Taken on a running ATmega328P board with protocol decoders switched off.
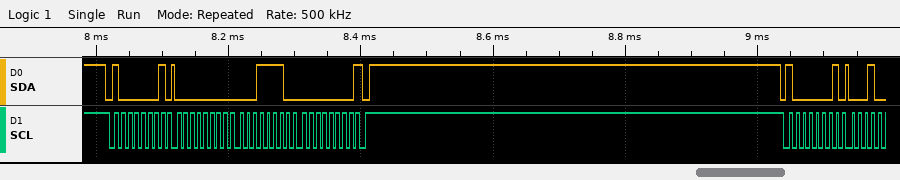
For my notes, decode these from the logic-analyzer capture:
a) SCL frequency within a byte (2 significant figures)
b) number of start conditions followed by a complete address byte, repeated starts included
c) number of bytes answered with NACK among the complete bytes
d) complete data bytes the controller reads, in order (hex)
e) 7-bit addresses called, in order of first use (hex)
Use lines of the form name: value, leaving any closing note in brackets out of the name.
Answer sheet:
SCL frequency within a byte: 100 kHz
number of start conditions followed by a complete address byte, repeated starts included: 2
number of bytes answered with NACK among the complete bytes: 1
complete data bytes the controller reads, in order: 00 1E 00
7-bit addresses called, in order of first use: 0x40
